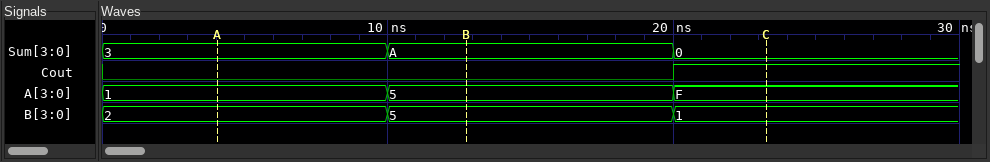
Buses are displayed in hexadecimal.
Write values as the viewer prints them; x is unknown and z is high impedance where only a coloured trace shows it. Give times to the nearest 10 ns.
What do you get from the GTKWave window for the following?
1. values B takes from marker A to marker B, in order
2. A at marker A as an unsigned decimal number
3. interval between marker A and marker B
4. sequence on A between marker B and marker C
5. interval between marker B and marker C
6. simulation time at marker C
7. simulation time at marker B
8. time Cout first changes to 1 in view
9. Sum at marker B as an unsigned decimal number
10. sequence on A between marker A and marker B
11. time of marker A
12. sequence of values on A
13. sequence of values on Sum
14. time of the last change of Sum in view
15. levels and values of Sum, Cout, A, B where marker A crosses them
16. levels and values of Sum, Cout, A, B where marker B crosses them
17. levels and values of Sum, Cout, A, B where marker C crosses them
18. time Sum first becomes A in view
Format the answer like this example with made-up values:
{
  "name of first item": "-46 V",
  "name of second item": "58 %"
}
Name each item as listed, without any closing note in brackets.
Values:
{
  "values B takes from marker A to marker B, in order": "2, 5",
  "A at marker A as an unsigned decimal number": "1",
  "interval between marker A and marker B": "10 ns",
  "sequence on A between marker B and marker C": "5, F",
  "interval between marker B and marker C": "10 ns",
  "simulation time at marker C": "20 ns",
  "simulation time at marker B": "10 ns",
  "time Cout first changes to 1 in view": "20 ns",
  "Sum at marker B as an unsigned decimal number": "10",
  "sequence on A between marker A and marker B": "1, 5",
  "time of marker A": "0 ns",
  "sequence of values on A": "1, 5, F",
  "sequence of values on Sum": "3, A, 0",
  "time of the last change of Sum in view": "20 ns",
  "levels and values of Sum, Cout, A, B where marker A crosses them": "Sum=3, Cout=0, A=1, B=2",
  "levels and values of Sum, Cout, A, B where marker B crosses them": "Sum=A, Cout=0, A=5, B=5",
  "levels and values of Sum, Cout, A, B where marker C crosses them": "Sum=0, Cout=1, A=F, B=1",
  "time Sum first becomes A in view": "10 ns"
}
